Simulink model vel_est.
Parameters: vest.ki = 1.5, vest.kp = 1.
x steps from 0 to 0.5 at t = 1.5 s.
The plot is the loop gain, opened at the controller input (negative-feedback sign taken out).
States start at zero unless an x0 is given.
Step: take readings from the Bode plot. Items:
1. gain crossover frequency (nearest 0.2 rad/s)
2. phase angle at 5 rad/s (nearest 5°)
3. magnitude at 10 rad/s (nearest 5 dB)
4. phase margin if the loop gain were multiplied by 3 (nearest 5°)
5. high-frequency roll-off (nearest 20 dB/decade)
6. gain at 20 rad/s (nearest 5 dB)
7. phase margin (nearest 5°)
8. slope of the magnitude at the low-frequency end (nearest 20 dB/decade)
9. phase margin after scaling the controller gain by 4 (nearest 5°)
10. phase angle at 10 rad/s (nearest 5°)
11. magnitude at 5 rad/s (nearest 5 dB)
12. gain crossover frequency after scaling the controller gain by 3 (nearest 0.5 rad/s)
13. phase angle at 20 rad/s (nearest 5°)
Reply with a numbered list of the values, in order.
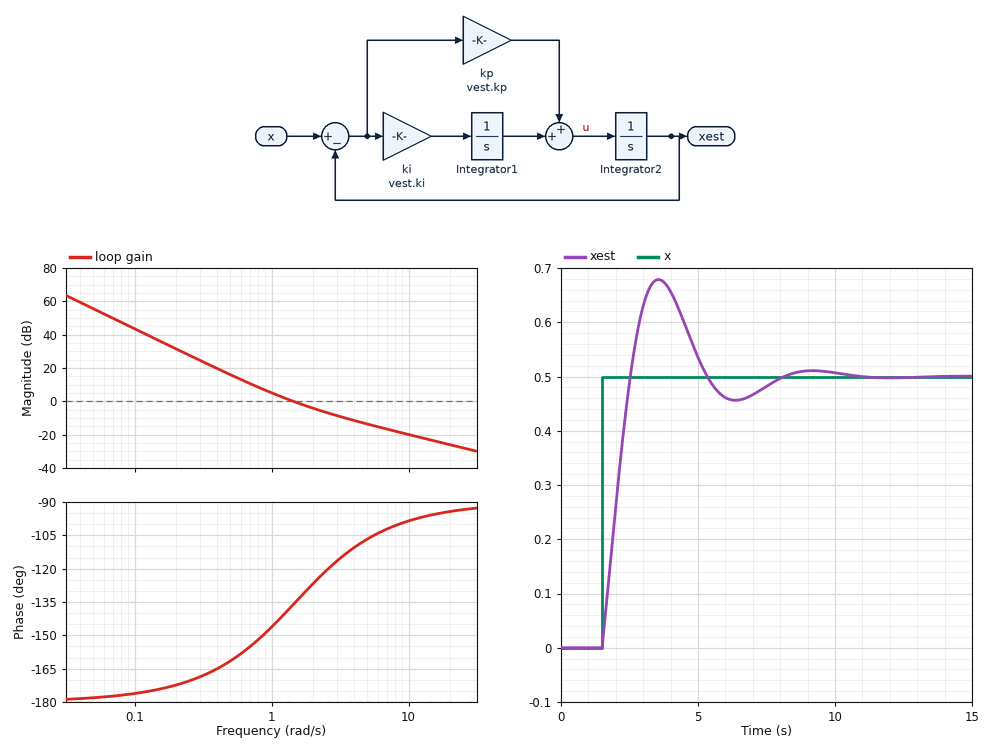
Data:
1. 1.4 rad/s
2. -105°
3. -20 dB
4. 65°
5. -20 dB/decade
6. -25 dB
7. 45°
8. -40 dB/decade
9. 70°
10. -100°
11. -15 dB
12. 3.5 rad/s
13. -95°
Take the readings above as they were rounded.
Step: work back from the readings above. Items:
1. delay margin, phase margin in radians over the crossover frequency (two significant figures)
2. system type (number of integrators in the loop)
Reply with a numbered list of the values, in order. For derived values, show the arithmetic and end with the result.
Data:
1. 45 × π / 180 / 1.4 = 0.56 s
2. 2
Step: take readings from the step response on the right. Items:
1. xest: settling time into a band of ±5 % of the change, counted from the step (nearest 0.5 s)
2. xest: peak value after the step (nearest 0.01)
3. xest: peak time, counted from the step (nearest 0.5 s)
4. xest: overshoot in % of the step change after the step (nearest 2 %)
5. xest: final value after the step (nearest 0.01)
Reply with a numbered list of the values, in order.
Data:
1. 6.0 s
2. 0.68
3. 2.0 s
4. 36 %
5. 0.50
